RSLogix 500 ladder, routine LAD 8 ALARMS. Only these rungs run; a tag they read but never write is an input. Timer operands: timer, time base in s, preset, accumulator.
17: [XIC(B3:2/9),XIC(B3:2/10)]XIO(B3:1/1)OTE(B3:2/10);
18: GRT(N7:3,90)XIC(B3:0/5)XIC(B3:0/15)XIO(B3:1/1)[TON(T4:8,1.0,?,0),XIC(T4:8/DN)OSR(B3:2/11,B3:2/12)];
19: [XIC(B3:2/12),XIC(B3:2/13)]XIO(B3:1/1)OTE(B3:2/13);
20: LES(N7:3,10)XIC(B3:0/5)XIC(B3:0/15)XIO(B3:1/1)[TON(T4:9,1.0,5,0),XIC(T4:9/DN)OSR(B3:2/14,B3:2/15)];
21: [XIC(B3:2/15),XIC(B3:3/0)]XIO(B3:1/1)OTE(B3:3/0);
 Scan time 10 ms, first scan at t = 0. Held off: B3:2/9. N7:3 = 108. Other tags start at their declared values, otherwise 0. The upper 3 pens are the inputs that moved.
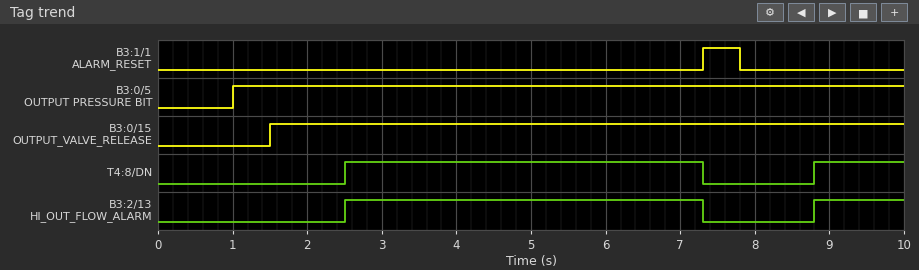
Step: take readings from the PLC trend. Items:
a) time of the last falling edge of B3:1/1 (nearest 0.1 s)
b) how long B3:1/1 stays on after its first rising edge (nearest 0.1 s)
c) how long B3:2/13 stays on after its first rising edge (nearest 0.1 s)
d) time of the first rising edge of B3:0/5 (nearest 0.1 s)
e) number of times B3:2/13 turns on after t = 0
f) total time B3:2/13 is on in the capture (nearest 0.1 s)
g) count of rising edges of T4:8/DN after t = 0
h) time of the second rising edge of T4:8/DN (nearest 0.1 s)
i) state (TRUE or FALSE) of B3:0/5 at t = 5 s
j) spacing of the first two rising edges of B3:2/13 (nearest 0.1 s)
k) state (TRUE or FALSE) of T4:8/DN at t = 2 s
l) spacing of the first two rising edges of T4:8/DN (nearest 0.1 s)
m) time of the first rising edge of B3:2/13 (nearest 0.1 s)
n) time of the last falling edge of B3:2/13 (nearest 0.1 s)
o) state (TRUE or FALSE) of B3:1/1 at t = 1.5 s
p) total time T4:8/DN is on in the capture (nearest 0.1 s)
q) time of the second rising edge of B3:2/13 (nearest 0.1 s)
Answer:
7.8 s
0.5 s
4.8 s
1.0 s
2
6.0 s
2
8.8 s
TRUE
6.3 s
FALSE
6.3 s
2.5 s
7.3 s
FALSE
6.0 s
8.8 s
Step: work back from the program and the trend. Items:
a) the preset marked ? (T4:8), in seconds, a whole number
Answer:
1 s
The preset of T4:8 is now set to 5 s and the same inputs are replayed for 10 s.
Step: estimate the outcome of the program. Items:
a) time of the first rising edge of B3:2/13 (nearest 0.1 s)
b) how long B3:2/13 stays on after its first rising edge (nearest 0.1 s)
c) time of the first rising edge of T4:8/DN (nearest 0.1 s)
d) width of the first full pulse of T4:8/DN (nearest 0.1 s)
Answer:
6.5 s
0.8 s
6.5 s
0.8 s
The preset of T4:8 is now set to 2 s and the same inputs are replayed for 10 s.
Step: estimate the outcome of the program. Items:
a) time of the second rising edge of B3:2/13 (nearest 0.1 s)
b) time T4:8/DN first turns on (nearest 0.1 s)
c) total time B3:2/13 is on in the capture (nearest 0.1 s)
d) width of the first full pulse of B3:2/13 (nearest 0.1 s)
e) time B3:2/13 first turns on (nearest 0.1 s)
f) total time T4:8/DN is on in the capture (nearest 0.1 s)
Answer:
9.8 s
3.5 s
4.0 s
3.8 s
3.5 s
4.0 s
